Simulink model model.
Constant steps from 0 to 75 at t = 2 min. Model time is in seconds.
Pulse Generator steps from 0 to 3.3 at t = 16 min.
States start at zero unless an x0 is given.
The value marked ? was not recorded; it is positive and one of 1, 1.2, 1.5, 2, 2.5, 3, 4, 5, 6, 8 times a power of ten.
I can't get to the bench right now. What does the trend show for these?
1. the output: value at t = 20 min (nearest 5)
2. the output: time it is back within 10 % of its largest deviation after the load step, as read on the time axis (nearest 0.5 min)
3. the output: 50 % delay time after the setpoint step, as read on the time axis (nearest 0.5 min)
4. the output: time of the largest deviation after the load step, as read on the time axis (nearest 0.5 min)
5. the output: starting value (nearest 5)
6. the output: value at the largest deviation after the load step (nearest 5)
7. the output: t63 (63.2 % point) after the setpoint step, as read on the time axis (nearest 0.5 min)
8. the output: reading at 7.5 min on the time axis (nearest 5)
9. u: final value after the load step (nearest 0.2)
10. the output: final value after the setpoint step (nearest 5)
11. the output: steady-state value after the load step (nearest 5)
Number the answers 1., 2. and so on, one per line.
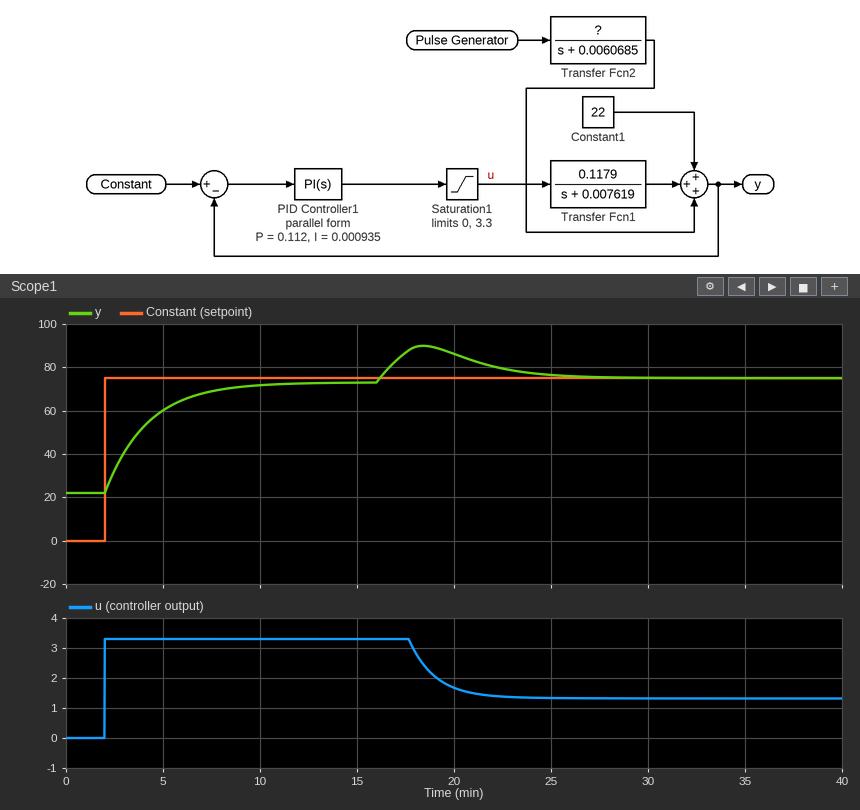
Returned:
1. 85
2. 24.5 min
3. 3.5 min
4. 18.5 min
5. 20
6. 90
7. 4.0 min
8. 70
9. 1.4
10. 75
11. 75
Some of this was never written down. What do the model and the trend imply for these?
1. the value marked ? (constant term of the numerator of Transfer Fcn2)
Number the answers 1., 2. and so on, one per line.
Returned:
1. 0.06
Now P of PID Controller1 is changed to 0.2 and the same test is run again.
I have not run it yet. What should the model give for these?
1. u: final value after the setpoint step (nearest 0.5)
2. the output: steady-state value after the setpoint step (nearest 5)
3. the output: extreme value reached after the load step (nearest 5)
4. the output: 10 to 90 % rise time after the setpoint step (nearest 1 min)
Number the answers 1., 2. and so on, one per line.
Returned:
1. 3.5
2. 75
3. 85
4. 5 min
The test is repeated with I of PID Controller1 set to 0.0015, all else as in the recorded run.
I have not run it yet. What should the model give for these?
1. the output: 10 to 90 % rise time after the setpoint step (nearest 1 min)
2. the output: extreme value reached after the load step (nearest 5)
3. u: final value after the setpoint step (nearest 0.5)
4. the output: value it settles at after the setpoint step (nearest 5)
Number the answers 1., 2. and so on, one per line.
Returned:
1. 5 min
2. 95
3. 3.5
4. 75
